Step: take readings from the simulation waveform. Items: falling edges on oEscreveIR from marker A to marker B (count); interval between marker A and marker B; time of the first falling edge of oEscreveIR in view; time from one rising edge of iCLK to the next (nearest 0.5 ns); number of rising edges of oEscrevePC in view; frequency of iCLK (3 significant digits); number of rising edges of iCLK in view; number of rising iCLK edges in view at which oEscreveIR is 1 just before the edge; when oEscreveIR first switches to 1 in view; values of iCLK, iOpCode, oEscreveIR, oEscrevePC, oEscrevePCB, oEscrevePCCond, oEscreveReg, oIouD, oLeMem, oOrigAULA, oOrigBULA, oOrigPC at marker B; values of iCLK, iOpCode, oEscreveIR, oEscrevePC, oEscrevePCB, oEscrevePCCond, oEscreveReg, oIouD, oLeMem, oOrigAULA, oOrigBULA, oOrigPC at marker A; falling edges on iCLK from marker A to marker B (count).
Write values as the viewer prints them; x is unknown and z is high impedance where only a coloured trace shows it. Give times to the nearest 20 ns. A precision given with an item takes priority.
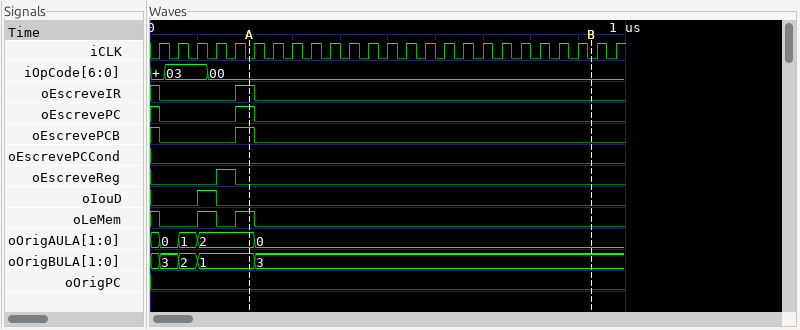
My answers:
1
720 ns
20 ns
40 ns
1
25.0 MHz
25
2
180 ns
iCLK=0, iOpCode=00, oEscreveIR=0, oEscrevePC=0, oEscrevePCB=0, oEscrevePCCond=0, oEscreveReg=0, oIouD=0, oLeMem=0, oOrigAULA=0, oOrigBULA=3, oOrigPC=0
iCLK=0, iOpCode=00, oEscreveIR=1, oEscrevePC=1, oEscrevePCB=1, oEscrevePCCond=0, oEscreveReg=0, oIouD=0, oLeMem=1, oOrigAULA=2, oOrigBULA=1, oOrigPC=0
18
